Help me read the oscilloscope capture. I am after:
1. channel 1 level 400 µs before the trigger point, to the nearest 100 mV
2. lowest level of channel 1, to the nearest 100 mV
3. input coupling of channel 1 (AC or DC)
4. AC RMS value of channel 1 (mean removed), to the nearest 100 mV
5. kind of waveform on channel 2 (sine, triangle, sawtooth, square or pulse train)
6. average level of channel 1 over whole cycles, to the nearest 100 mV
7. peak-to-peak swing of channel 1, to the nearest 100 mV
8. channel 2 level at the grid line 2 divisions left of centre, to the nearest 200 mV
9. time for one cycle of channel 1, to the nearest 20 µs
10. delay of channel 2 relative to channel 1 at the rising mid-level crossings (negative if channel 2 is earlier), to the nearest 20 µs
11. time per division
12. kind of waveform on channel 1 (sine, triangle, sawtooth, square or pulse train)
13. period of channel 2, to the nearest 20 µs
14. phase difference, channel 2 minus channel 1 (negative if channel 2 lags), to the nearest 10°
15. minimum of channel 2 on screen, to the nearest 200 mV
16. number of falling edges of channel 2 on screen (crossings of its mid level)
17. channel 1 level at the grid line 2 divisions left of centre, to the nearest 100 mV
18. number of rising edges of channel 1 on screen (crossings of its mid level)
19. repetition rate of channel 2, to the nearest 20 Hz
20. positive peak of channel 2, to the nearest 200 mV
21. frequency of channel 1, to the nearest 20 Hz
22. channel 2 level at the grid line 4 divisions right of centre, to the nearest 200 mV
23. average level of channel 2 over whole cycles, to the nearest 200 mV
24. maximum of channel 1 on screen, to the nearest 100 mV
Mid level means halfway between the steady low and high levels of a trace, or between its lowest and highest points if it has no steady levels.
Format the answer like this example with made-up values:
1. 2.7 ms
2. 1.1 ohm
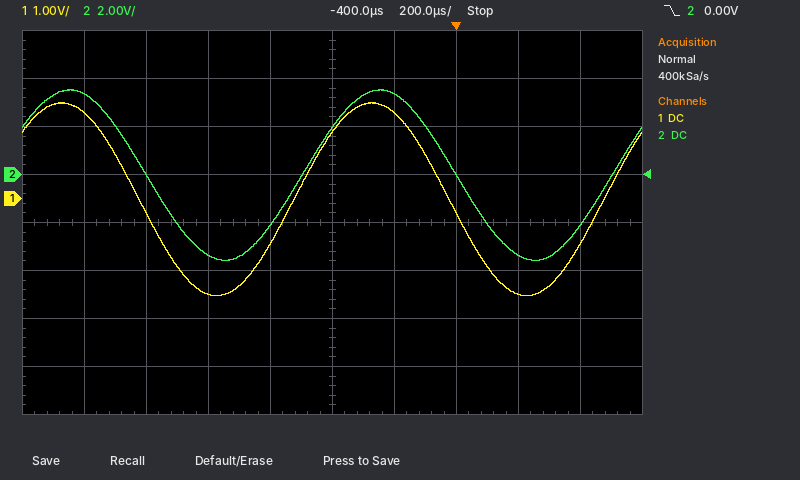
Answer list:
1. 1.4 V
2. -2.0 V
3. DC
4. 1.4 V
5. sine
6. 0.0 V
7. 4.0 V
8. -3.4 V
9. 1.00 ms
10. +20 µs
11. 200 µs
12. sine
13. 1.00 ms
14. -10°
15. -3.6 V
16. 2
17. -2.0 V
18. 2
19. 1.00 kHz
20. 3.6 V
21. 1.00 kHz
22. -2.2 V
23. 0.0 V
24. 2.0 V
